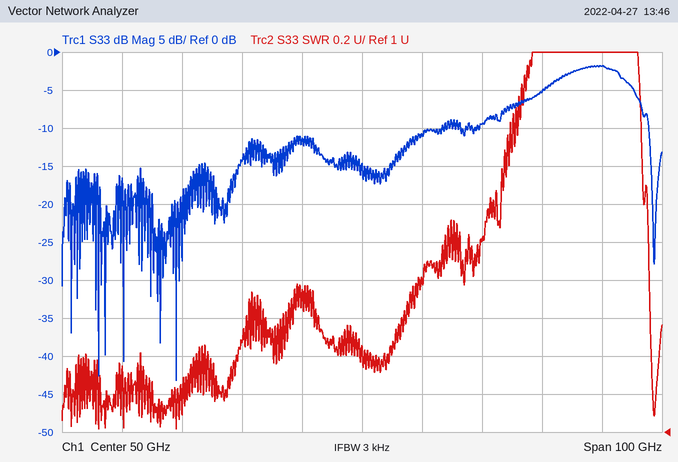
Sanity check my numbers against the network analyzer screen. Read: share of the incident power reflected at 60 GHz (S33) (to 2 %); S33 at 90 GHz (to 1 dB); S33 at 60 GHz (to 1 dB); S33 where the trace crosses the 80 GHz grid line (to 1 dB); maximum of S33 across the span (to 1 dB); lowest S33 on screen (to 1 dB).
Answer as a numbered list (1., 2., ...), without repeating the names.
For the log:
1. 8 %
2. -2 dB
3. -11 dB
4. -5 dB
5. -2 dB
6. -43 dB
